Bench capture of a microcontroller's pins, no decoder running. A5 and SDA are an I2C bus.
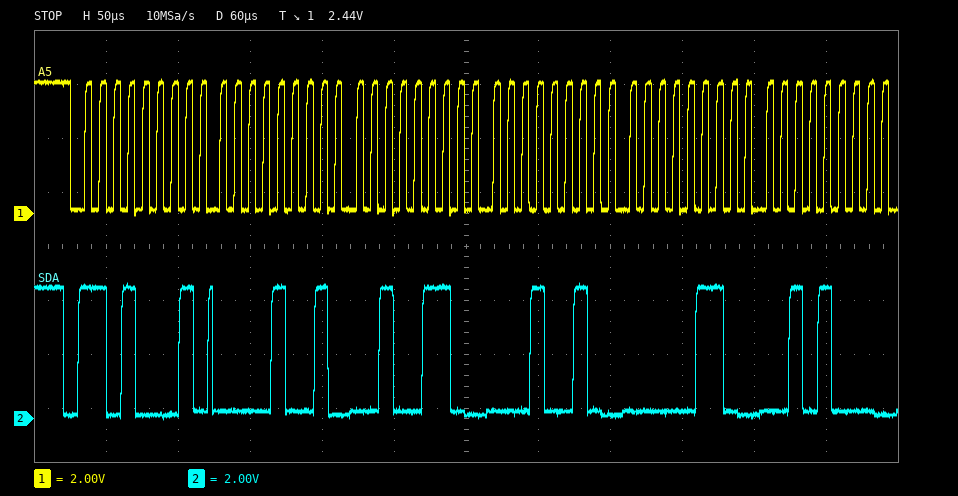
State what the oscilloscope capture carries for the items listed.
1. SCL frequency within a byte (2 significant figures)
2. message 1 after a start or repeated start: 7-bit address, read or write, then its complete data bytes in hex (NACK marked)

100 kHz
0x68 read: 09 26 12 06 28
